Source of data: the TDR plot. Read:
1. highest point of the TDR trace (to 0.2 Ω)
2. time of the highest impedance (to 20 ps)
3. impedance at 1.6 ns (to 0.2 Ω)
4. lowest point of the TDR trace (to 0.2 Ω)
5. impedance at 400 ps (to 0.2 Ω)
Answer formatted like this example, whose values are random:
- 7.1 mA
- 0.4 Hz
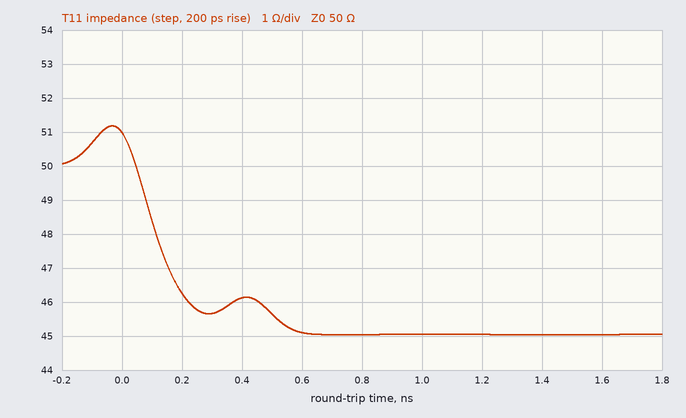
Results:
- 51.2 Ω
- -40 ps
- 45.0 Ω
- 45.0 Ω
- 46.2 Ω
